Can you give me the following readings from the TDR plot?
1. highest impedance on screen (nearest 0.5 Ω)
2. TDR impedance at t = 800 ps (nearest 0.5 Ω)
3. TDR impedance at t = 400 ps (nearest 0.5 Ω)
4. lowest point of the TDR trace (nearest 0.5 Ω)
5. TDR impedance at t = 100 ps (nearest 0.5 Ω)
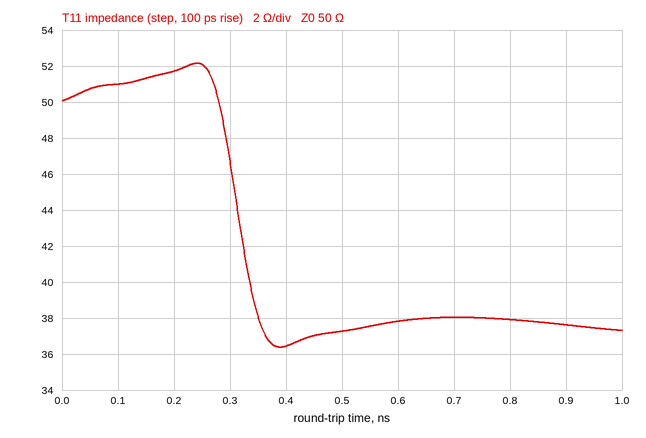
52.0 Ω
38.0 Ω
36.5 Ω
36.5 Ω
51.0 Ω
